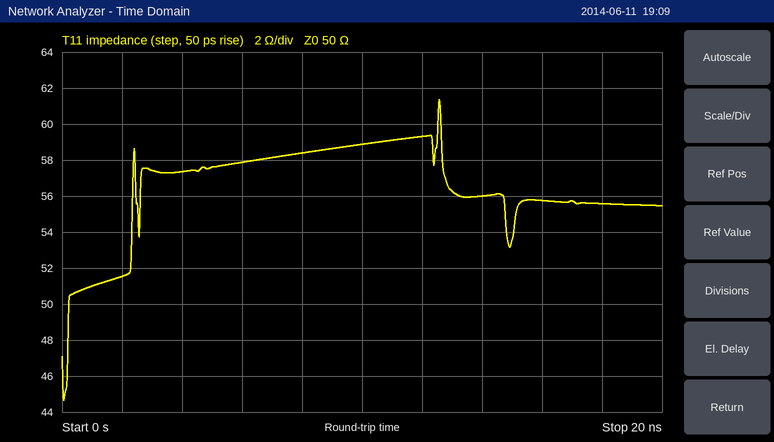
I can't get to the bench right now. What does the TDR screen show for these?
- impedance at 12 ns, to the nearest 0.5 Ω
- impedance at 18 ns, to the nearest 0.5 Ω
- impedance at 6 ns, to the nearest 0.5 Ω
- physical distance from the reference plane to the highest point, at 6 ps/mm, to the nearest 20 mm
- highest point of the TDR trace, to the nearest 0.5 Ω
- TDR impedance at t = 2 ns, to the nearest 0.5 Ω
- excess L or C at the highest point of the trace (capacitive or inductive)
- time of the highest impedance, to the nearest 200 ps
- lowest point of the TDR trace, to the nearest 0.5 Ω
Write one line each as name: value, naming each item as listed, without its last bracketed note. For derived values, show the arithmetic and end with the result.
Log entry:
impedance at 12 ns, to the nearest 0.5 Ω: 59.5 Ω
impedance at 18 ns, to the nearest 0.5 Ω: 55.5 Ω
impedance at 6 ns, to the nearest 0.5 Ω: 58.0 Ω
physical distance from the reference plane to the highest point, at 6 ps/mm, to the nearest 20 mm: 12.6 ns / 2 / 6 ps/mm ≈ 1.05 m, so 1.04 m to the nearest 20 mm
highest point of the TDR trace, to the nearest 0.5 Ω: 61.5 Ω
TDR impedance at t = 2 ns, to the nearest 0.5 Ω: 51.5 Ω
excess L or C at the highest point of the trace: inductive
time of the highest impedance, to the nearest 200 ps: 12.6 ns
lowest point of the TDR trace, to the nearest 0.5 Ω: 44.5 Ω
